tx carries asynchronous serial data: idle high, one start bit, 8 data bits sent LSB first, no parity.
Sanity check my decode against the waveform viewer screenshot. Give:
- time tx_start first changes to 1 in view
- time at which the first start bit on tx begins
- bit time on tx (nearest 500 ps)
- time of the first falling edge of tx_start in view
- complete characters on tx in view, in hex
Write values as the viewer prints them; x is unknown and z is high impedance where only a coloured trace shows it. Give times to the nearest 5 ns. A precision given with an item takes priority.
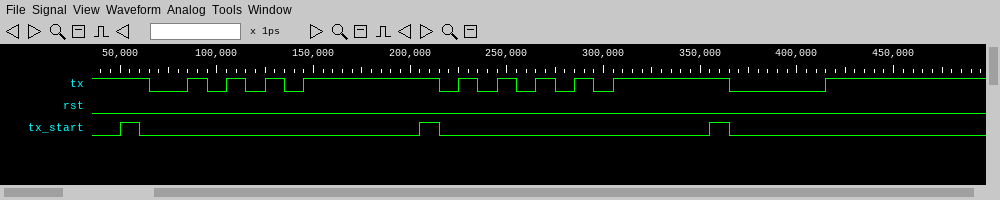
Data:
50 ns
65 ns
10000 ps
60 ns
AA, 55, F0
